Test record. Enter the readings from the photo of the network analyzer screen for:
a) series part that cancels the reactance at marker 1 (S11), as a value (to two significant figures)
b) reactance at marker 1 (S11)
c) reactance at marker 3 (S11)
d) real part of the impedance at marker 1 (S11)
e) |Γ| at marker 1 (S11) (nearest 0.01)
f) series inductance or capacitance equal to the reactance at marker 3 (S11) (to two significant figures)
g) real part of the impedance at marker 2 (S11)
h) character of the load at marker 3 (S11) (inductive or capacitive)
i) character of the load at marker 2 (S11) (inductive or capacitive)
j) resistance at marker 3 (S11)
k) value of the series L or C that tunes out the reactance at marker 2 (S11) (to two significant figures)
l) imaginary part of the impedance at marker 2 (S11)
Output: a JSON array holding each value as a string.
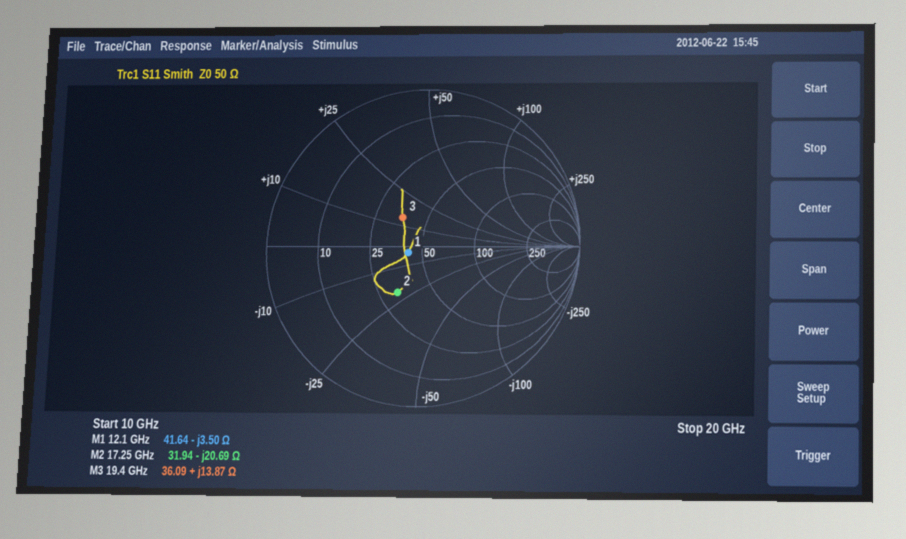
["46 pH", "-3.50 Ω", "+13.87 Ω", "41.64 Ω", "0.10", "110 pH", "31.94 Ω", "inductive", "capacitive", "36.09 Ω", "190 pH", "-20.69 Ω"]
